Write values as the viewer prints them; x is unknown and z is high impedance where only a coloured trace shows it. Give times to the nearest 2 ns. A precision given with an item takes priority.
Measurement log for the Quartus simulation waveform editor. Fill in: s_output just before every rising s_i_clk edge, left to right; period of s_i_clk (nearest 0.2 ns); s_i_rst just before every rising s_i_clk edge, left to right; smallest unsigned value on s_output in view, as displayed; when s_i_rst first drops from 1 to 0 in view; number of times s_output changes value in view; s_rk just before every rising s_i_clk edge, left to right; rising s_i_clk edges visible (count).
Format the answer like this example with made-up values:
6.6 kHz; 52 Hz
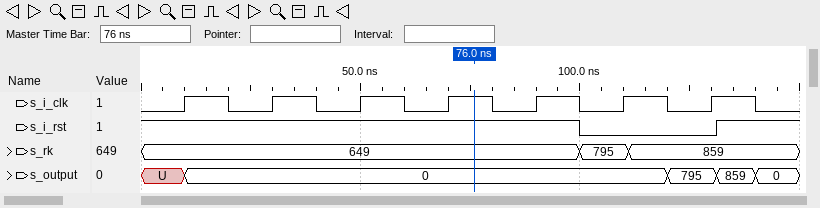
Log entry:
U, 0, 0, 0, 0, 0, 795; 20 ns; 1 1 1 1 1 0 0; 0; 100 ns; 4; 649, 649, 649, 649, 649, 795, 859; 7
